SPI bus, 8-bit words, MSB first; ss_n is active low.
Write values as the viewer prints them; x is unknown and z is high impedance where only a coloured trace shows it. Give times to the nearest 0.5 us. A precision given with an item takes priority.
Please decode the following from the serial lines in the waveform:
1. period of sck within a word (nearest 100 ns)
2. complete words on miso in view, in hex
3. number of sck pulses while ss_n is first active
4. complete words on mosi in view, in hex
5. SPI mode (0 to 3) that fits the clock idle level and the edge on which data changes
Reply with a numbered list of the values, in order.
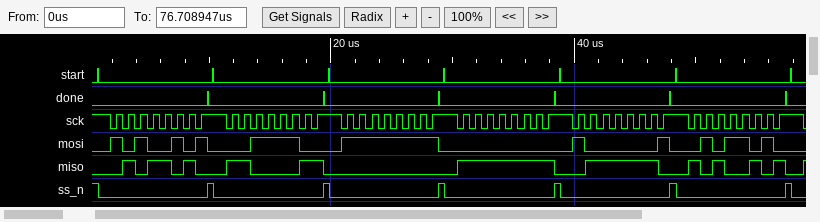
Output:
1. 1000 ns
2. 5A, C3, 00, FF, 7E, A5
3. 8
4. A5, 3C, FF, 00, 81, 5A
5. 3
